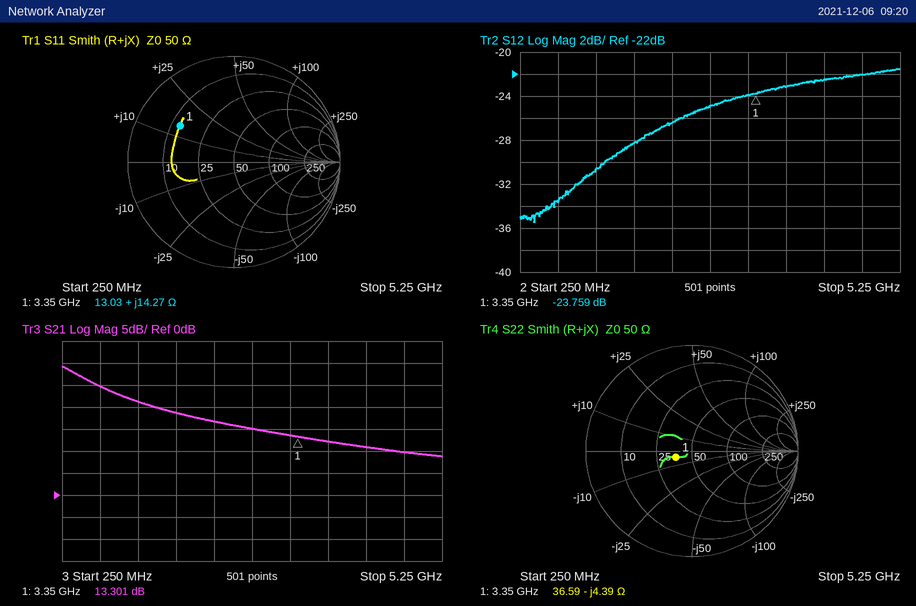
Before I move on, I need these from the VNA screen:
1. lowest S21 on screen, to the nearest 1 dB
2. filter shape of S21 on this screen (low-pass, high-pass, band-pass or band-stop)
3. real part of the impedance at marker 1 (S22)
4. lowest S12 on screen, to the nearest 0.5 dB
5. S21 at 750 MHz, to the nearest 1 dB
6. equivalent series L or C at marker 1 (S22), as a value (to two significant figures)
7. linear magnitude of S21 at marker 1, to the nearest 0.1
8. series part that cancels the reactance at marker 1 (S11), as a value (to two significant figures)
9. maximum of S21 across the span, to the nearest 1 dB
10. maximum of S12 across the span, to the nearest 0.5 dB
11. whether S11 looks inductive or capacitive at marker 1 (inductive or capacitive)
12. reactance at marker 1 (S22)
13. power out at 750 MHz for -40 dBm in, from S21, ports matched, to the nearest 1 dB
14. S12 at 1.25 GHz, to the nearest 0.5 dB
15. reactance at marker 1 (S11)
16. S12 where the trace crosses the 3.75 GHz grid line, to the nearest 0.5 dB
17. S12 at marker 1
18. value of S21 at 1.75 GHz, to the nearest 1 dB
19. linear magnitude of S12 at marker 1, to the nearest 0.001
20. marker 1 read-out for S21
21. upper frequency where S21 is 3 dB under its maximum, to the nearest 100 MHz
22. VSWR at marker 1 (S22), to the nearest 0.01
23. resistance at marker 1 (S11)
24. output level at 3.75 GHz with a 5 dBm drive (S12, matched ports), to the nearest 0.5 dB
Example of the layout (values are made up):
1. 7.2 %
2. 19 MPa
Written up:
1. 9 dB
2. low-pass
3. 36.59 Ω
4. -35.5 dB
5. 25 dB
6. 11 pF
7. 4.6
8. 3.3 pF
9. 29 dB
10. -21.5 dB
11. inductive
12. -4.39 Ω
13. -15 dBm
14. -30.5 dB
15. +14.27 Ω
16. -23.0 dB
17. -23.759 dB
18. 19 dB
19. 0.065
20. 13.301 dB
21. 600 MHz
22. 1.39
23. 13.03 Ω
24. -18.0 dBm
